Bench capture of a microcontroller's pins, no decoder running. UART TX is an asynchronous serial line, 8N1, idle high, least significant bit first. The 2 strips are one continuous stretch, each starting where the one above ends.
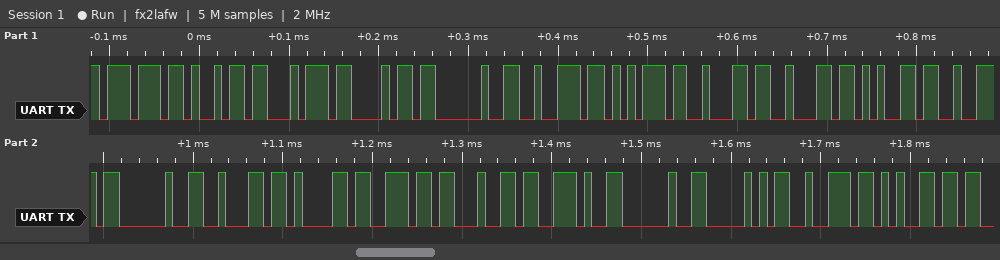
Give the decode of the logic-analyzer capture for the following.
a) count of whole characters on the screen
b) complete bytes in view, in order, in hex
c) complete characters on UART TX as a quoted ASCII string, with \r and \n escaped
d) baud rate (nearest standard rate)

21
77 69 74 68 20 72 75 62 62 65 72 20 62 61 6E 64 2E 20 50 72 65
"with rubber band. Pre"
115200 baud
